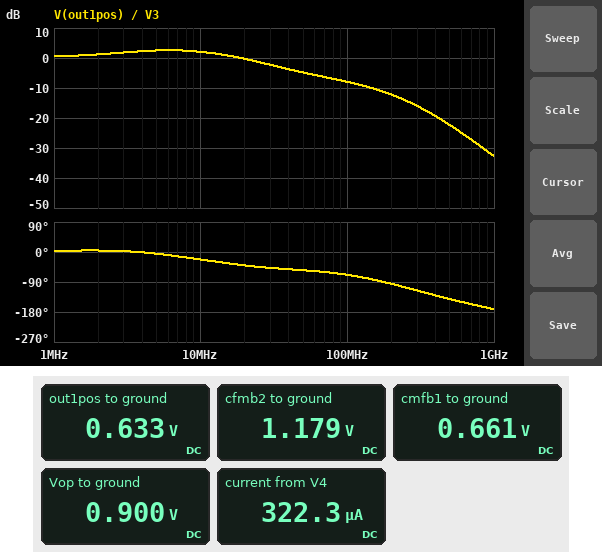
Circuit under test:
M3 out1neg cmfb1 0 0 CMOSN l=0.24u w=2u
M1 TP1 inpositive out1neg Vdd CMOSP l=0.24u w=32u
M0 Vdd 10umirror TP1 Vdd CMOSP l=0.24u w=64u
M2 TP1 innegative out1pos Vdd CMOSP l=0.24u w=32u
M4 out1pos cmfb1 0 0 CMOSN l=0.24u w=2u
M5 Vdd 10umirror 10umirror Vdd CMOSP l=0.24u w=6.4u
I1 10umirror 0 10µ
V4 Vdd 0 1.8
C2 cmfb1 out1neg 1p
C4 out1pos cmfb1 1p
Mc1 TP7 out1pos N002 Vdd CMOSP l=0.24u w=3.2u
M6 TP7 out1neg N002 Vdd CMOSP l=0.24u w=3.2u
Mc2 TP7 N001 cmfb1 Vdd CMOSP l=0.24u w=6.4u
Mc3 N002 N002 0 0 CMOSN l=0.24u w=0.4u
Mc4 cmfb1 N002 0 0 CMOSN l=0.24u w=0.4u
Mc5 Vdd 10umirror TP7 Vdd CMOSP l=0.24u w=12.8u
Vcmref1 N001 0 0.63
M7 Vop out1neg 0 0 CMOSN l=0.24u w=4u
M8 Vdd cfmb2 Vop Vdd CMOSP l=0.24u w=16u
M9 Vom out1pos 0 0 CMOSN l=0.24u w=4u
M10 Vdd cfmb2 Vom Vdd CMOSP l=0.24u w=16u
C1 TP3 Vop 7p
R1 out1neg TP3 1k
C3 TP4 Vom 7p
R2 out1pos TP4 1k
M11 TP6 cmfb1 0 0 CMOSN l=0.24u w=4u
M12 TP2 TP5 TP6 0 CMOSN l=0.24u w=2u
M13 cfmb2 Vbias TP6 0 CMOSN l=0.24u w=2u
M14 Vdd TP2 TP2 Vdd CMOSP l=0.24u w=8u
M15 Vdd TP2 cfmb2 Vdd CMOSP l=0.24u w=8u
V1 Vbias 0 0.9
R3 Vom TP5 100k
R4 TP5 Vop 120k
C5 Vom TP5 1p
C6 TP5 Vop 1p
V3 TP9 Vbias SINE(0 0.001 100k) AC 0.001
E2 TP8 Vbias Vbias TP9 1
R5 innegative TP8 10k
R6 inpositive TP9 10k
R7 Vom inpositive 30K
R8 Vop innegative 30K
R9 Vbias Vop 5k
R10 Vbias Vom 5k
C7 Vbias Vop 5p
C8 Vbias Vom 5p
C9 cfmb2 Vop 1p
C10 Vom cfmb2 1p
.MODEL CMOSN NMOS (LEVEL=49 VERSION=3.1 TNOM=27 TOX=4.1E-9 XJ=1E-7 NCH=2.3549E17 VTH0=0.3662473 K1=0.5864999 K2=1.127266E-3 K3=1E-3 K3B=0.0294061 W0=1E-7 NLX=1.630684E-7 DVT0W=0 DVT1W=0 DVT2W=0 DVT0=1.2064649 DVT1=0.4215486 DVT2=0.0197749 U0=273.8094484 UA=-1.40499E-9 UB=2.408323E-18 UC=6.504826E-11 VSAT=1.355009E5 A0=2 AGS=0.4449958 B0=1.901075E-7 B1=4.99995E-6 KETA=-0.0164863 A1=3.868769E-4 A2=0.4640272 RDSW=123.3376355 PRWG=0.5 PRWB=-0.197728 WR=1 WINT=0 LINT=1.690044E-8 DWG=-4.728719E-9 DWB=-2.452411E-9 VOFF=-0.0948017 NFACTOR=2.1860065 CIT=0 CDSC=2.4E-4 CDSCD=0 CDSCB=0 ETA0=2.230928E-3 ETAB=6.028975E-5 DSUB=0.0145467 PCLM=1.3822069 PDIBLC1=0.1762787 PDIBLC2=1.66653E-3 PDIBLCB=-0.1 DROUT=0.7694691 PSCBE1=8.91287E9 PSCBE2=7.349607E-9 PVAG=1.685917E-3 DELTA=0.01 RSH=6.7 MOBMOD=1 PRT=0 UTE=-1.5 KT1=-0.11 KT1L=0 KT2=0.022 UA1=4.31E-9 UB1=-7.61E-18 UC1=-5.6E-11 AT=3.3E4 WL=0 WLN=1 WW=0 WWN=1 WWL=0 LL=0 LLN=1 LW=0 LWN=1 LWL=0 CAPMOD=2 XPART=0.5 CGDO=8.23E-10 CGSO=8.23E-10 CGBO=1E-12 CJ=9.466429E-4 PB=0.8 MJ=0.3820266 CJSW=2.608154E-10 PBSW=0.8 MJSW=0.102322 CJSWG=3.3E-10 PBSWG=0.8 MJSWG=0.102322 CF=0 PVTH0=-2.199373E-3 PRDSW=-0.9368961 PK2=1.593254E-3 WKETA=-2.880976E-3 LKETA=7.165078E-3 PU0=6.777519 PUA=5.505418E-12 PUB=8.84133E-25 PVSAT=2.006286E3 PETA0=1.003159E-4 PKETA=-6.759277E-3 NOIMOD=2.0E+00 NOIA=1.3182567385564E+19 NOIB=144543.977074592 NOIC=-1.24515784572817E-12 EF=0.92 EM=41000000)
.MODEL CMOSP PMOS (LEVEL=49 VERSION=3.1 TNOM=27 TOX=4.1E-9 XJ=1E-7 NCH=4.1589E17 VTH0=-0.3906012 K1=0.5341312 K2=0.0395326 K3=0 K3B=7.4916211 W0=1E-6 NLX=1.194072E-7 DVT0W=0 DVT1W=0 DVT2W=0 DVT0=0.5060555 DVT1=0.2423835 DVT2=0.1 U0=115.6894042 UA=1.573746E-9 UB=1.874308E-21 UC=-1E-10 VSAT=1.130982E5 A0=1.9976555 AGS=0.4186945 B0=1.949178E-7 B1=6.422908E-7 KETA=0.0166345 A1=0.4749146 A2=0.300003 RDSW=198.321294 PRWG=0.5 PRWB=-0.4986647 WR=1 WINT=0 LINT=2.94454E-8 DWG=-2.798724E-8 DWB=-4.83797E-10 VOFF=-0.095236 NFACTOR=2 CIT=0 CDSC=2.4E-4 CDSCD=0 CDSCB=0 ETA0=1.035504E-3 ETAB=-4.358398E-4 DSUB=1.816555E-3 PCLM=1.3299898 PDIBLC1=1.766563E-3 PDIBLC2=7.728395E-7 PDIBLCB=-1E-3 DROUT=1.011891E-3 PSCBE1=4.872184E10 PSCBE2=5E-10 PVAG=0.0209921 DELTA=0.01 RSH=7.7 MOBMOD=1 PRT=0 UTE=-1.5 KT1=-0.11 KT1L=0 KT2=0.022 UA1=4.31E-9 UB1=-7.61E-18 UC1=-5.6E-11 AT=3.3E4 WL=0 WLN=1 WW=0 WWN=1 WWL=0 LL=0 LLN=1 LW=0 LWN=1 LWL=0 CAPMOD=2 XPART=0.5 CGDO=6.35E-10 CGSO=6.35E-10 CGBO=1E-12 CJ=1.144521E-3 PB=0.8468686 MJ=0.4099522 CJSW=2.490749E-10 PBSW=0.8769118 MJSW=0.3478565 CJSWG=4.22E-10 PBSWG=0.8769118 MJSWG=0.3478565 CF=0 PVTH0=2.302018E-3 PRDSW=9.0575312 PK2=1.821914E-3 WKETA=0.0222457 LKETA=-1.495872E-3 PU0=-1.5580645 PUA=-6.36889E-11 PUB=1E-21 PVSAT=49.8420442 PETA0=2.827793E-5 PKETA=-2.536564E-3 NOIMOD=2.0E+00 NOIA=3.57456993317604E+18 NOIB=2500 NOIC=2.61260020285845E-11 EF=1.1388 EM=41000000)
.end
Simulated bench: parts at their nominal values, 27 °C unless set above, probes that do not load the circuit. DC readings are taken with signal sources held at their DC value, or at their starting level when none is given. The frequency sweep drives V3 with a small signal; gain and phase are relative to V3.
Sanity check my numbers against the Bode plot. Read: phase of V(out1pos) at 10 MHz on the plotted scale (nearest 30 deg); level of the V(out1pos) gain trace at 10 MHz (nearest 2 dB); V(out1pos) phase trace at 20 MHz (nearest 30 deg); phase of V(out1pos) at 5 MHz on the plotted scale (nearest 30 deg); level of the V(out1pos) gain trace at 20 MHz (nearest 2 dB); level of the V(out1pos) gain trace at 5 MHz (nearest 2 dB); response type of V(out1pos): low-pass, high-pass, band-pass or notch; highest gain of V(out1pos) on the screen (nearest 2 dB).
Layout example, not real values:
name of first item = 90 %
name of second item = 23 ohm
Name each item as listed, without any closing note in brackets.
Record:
phase of V(out1pos) at 10 MHz on the plotted scale = -30 deg
level of the V(out1pos) gain trace at 10 MHz = 2 dB
V(out1pos) phase trace at 20 MHz = -30 deg
phase of V(out1pos) at 5 MHz on the plotted scale = 0 deg
level of the V(out1pos) gain trace at 20 MHz = 0 dB
level of the V(out1pos) gain trace at 5 MHz = 2 dB
response type of V(out1pos): low-pass, high-pass, band-pass or notch = low-pass
highest gain of V(out1pos) on the screen = 2 dB
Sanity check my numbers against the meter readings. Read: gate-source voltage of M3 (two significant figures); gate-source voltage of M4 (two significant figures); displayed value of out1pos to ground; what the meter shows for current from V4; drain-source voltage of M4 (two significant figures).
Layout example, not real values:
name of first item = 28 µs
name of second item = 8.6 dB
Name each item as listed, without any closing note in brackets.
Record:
gate-source voltage of M3 = 660 mV
gate-source voltage of M4 = 660 mV
displayed value of out1pos to ground = 0.633 V
what the meter shows for current from V4 = 322.3 µA
drain-source voltage of M4 = 630 mV
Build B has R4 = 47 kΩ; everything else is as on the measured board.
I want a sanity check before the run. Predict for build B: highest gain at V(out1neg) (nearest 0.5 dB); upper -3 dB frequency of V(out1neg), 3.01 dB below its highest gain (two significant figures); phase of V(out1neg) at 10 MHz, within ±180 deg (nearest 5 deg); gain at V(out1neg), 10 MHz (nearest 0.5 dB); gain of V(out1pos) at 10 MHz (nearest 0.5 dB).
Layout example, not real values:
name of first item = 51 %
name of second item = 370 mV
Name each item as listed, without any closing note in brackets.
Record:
highest gain at V(out1neg) = 3.0 dB
upper -3 dB frequency of V(out1neg), 3.01 dB below its highest gain = 19 MHz
phase of V(out1neg) at 10 MHz, within ±180 deg = 155 deg
gain at V(out1neg), 10 MHz = 1.5 dB
gain of V(out1pos) at 10 MHz = 2.5 dB
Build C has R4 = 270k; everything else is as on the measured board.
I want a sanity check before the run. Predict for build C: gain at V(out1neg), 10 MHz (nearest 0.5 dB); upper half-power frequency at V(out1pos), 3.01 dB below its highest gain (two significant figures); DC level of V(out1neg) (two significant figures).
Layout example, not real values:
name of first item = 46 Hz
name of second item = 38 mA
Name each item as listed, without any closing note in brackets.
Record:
gain at V(out1neg), 10 MHz = 2.5 dB
upper half-power frequency at V(out1pos), 3.01 dB below its highest gain = 20 MHz
DC level of V(out1neg) = 630 mV
